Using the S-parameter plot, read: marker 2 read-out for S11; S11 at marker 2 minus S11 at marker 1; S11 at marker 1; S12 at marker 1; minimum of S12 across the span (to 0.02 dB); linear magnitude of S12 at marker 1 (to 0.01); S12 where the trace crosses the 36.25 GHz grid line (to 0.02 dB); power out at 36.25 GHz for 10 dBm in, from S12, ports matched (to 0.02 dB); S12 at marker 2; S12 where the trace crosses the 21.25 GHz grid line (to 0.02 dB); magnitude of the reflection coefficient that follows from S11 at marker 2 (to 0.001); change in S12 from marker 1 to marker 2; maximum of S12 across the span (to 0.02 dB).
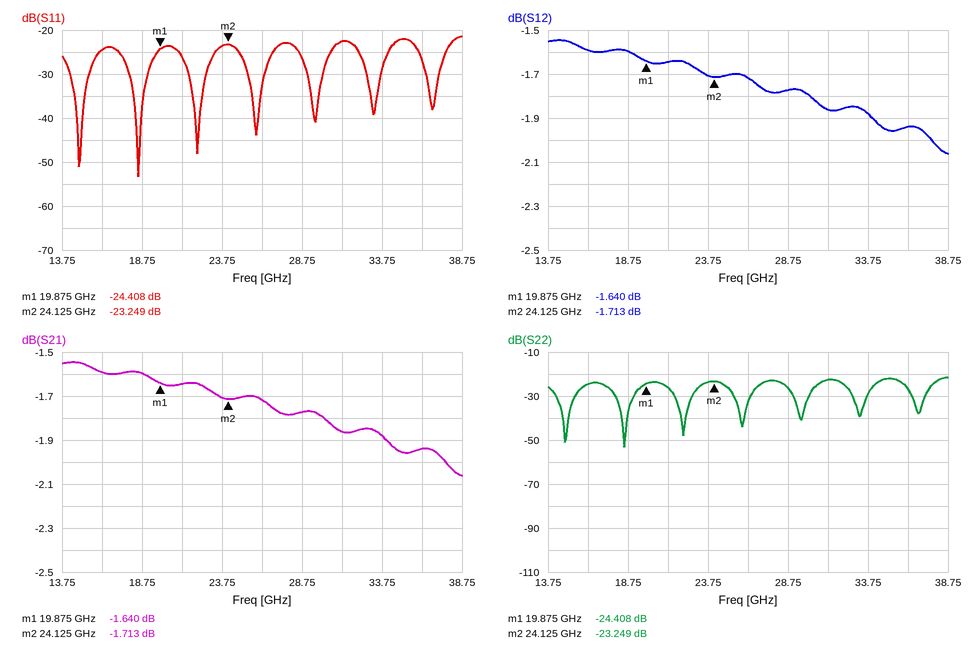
-23.249 dB
1.159 dB
-24.408 dB
-1.640 dB
-2.06 dB
0.83
-1.94 dB
8.06 dBm
-1.713 dB
-1.64 dB
0.069
-0.073 dB
-1.54 dB
